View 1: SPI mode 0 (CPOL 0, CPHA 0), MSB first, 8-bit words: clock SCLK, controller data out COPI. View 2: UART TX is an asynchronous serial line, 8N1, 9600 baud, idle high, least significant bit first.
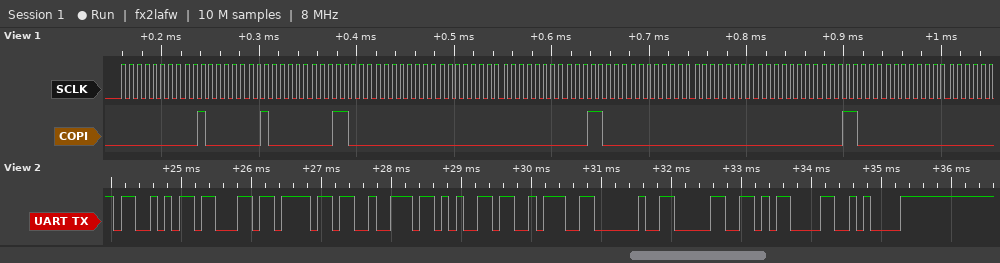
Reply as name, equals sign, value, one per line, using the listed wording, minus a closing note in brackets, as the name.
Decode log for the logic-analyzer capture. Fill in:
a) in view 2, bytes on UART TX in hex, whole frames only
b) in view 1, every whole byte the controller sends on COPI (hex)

in view 2, bytes on UART TX in hex, whole frames only = 53 63 6F 72 65 3A 20 30 0D 0A
in view 1, every whole byte the controller sends on COPI = 00 20 20 18 00 00 00 18 00 00 00 18 00
